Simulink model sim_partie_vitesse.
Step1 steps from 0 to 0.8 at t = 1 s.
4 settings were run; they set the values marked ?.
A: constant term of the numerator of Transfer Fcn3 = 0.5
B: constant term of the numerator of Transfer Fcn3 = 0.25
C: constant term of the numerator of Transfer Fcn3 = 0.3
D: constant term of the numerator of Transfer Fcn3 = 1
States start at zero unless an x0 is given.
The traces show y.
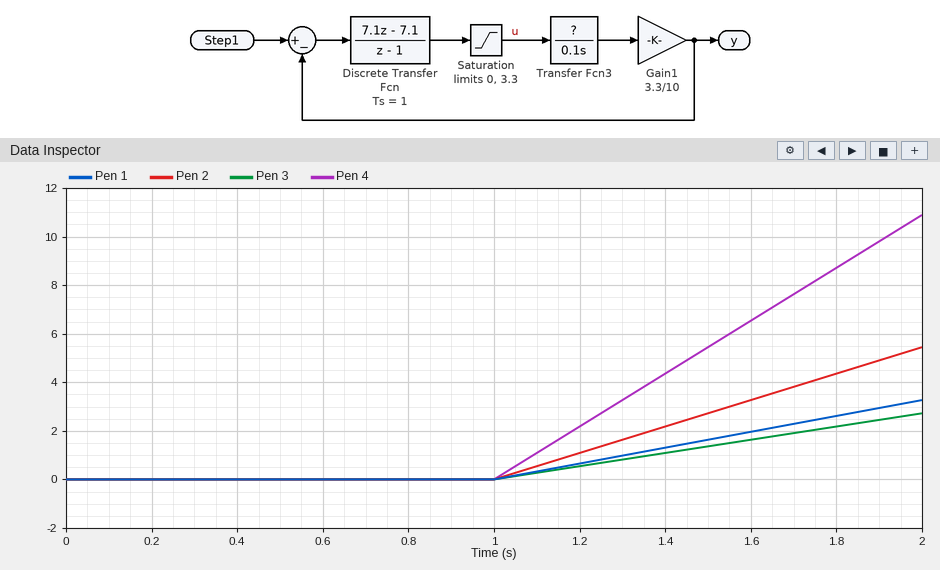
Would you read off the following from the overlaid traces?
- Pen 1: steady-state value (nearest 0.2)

3.2
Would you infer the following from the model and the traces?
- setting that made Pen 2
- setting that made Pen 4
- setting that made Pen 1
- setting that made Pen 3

A
D
C
B
